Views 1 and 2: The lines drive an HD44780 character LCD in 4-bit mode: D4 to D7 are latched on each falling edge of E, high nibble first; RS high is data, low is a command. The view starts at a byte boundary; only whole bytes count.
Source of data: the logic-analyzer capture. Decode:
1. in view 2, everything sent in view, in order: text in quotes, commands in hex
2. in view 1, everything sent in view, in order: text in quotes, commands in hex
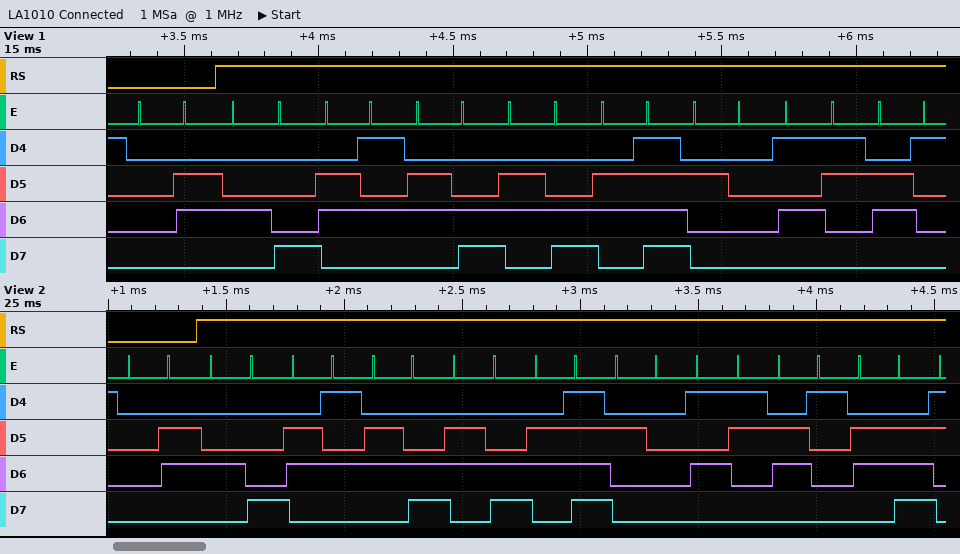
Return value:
0x06 "Hello San"
0x06 "Hello Sa"
